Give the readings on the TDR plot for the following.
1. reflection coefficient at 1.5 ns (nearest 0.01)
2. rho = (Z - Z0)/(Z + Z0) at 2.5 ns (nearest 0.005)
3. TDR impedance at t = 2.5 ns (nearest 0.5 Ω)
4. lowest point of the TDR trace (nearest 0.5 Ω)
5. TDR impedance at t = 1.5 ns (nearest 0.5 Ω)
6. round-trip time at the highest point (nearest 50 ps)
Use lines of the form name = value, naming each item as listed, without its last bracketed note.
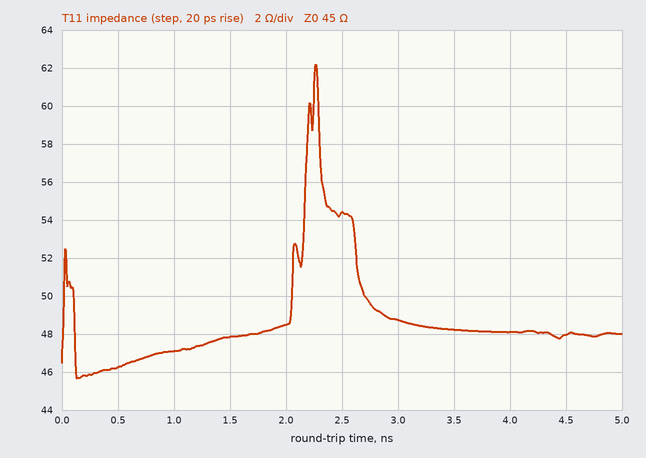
reflection coefficient at 1.5 ns = +0.03
rho = (Z - Z0)/(Z + Z0) at 2.5 ns = +0.095
TDR impedance at t = 2.5 ns = 54.5 Ω
lowest point of the TDR trace = 45.5 Ω
TDR impedance at t = 1.5 ns = 48.0 Ω
round-trip time at the highest point = 2.25 ns
